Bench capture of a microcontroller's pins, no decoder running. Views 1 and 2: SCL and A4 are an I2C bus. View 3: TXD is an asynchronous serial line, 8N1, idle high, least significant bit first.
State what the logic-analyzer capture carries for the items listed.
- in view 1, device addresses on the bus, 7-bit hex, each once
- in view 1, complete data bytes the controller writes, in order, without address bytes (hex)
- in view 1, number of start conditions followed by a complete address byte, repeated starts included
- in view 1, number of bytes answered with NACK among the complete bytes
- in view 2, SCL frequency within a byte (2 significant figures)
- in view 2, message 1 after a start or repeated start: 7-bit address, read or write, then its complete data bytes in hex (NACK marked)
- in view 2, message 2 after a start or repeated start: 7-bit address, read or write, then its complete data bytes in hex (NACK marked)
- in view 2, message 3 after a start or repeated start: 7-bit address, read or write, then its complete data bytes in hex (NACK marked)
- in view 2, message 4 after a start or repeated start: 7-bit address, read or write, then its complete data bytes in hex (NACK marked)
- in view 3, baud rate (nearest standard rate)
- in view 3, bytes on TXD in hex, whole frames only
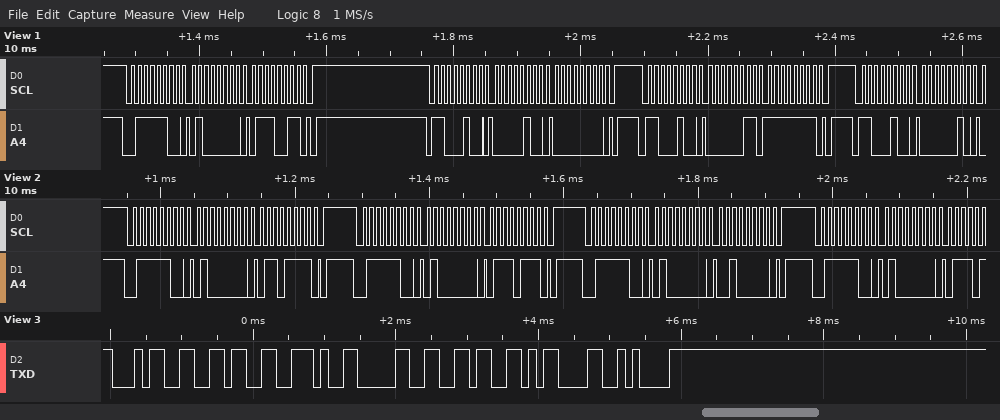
0x3E 0x62
40 73 04 00 03 FF 02
4
0
100 kHz
0x3E write: 40 6F
0x3E write: 40 77
0x3E write: 40 20
0x3E write: 40
9600 baud
34 36 2E 30 36 0D 0A
